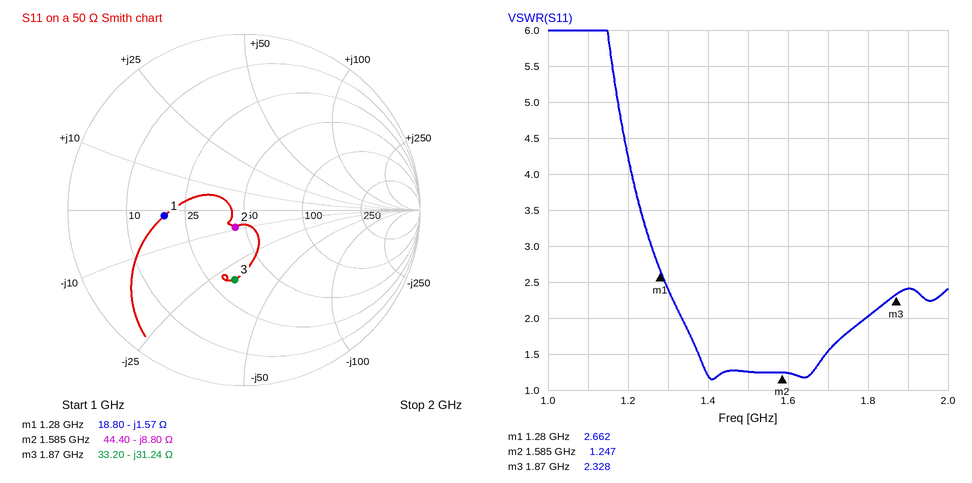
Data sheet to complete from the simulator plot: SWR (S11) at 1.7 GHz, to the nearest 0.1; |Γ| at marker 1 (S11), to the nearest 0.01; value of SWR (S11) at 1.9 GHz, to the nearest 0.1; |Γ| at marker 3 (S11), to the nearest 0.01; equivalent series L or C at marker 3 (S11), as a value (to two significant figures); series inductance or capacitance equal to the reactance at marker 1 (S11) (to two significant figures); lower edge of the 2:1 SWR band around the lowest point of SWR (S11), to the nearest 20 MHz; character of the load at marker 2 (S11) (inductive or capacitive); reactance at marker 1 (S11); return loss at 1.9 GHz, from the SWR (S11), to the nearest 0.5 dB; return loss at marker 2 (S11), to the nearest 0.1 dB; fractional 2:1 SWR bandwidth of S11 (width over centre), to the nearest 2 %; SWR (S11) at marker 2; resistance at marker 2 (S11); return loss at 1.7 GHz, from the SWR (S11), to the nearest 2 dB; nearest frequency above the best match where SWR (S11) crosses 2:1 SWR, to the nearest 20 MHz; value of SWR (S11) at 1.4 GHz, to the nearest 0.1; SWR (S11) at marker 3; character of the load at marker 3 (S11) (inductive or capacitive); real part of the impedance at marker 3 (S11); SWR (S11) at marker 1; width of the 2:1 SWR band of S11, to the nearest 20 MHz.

1.5
0.45
2.4
0.40
2.7 pF
79 pF
1.34 GHz
capacitive
-1.57 Ω
7.5 dB
19.2 dB
30 %
1.247
44.40 Ω
14 dB
1.80 GHz
1.2
2.328
capacitive
33.20 Ω
2.662
460 MHz
